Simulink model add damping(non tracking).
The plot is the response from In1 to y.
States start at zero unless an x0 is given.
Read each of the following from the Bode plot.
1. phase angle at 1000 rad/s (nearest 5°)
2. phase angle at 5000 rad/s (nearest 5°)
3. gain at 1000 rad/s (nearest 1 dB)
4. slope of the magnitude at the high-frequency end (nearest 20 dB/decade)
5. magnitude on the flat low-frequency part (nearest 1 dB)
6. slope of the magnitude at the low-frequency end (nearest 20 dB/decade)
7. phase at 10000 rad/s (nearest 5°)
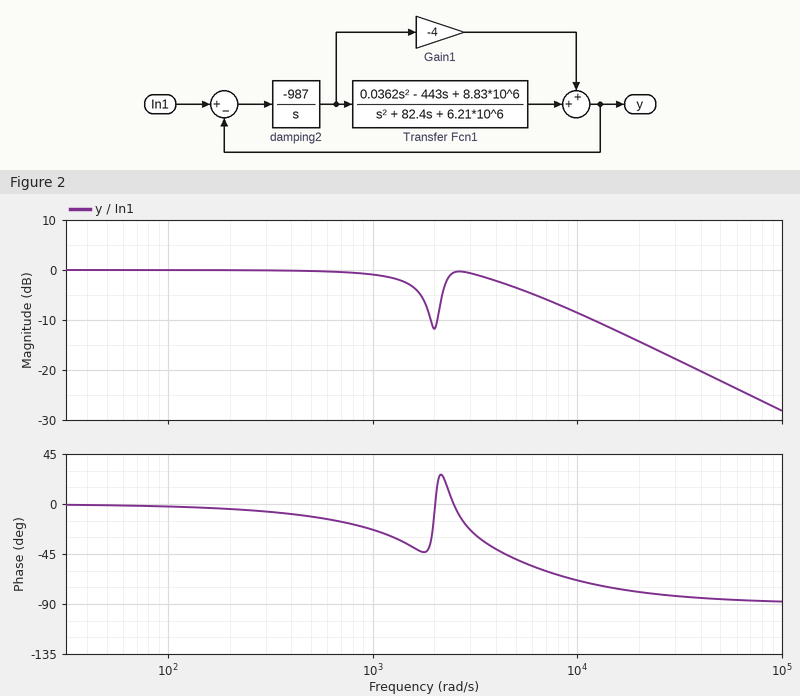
-25°
-50°
-1 dB
-20 dB/decade
0 dB
0 dB/decade
-70°
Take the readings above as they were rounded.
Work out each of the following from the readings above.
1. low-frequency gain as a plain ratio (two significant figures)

1.0
